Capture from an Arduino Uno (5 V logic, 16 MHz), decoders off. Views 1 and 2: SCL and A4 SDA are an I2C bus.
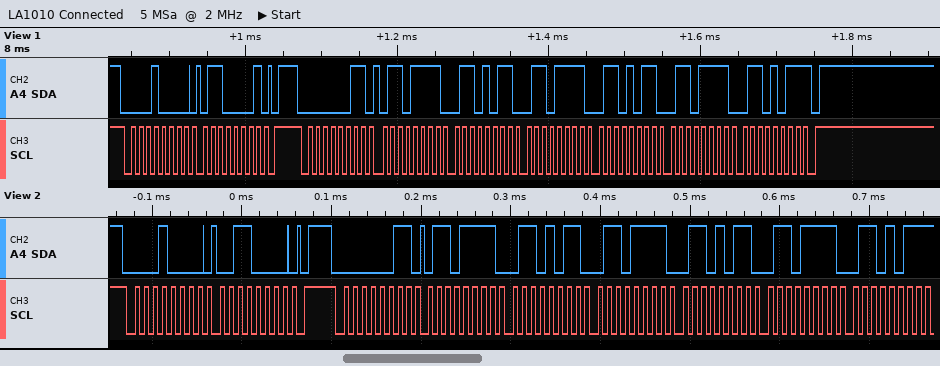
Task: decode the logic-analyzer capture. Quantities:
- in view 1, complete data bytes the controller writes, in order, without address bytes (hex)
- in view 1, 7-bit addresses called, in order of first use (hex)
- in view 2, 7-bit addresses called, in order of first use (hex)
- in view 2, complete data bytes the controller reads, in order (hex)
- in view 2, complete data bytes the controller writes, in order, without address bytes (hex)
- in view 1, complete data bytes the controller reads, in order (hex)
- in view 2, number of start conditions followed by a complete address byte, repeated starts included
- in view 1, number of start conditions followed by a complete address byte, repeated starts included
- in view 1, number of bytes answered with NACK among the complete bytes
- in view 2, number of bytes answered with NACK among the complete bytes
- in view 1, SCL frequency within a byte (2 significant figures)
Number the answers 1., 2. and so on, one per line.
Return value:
1. 61
2. 0x08 0x01
3. 0x08 0x01
4. 6F 6B 6F 6B 6F 6B
5. 30
6. 6F 6B 6F 6B 6F 6B
7. 2
8. 2
9. 1
10. 1
11. 100 kHz
